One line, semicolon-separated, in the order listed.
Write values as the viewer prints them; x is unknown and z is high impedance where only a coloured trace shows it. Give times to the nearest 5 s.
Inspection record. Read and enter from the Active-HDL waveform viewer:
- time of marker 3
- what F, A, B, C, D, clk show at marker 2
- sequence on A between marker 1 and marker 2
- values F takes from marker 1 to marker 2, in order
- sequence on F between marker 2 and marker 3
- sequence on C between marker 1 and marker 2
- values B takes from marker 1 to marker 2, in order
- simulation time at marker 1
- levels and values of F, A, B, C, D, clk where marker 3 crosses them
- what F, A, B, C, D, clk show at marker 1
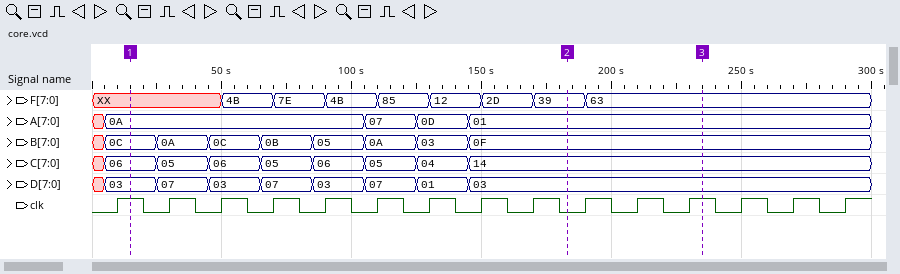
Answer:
235 s; F=39, A=01, B=0F, C=14, D=03, clk=0; 0A, 07, 0D, 01; XX, 4B, 7E, 4B, 85, 12, 2D, 39; 39, 63; 06, 05, 06, 05, 06, 05, 04, 14; 0C, 0A, 0C, 0B, 05, 0A, 03, 0F; 15 s; F=63, A=01, B=0F, C=14, D=03, clk=1; F=XX, A=0A, B=0C, C=06, D=03, clk=1
